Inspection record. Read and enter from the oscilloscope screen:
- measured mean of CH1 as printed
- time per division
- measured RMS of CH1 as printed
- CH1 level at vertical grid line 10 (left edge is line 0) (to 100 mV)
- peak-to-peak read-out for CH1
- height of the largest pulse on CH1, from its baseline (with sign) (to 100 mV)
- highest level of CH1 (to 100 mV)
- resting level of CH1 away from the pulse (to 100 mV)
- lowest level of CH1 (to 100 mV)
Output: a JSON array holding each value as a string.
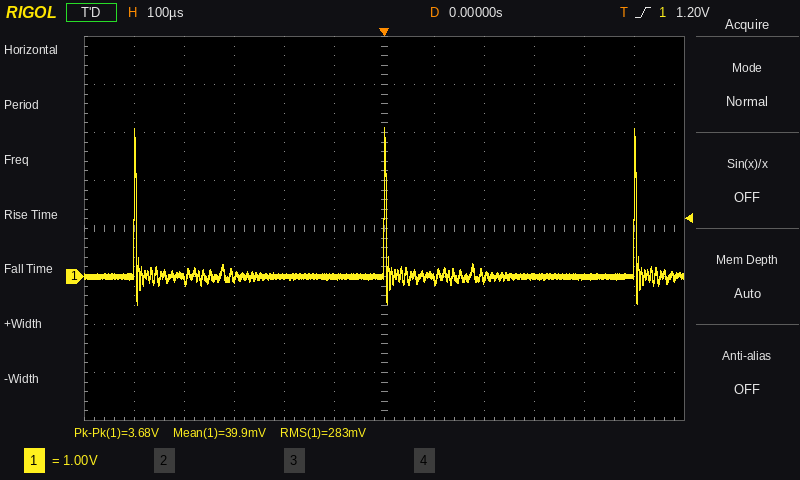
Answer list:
["39.9 mV", "100 µs", "283 mV", "0.0 V", "3.68 V", "+3.1 V", "3.1 V", "0.0 V", "-600 mV"]
